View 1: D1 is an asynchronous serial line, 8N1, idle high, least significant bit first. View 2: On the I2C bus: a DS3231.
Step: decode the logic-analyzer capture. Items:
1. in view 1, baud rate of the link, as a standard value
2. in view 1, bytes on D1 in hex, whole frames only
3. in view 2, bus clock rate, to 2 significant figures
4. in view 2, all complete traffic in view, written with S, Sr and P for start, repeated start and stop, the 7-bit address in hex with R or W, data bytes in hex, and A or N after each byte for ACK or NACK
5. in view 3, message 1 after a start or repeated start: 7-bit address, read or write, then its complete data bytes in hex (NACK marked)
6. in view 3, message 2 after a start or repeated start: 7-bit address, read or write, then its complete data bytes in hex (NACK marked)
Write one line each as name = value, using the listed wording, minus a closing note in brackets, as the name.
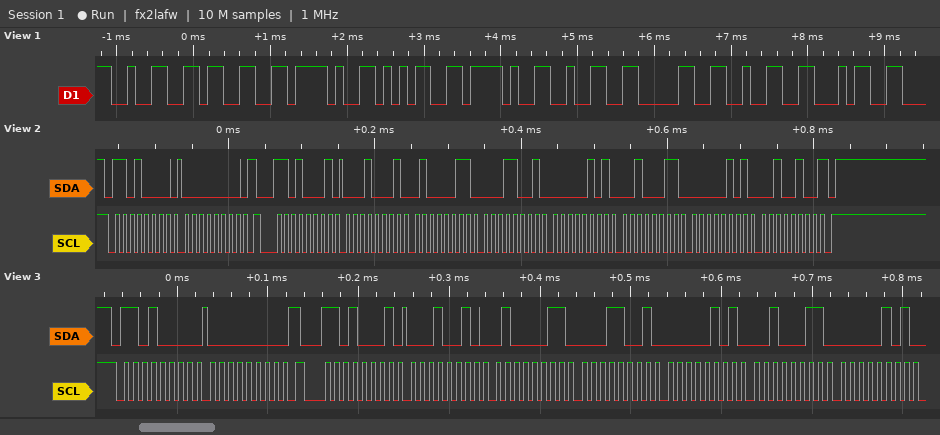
in view 1, baud rate of the link, as a standard value = 9600 baud
in view 1, bytes on D1 in hex, whole frames only = 0x32 0x33 0x2F 0x35 0x2F 0x32 0x30 0x32 0x34
in view 2, bus clock rate, to 2 significant figures = 100 kHz
in view 2, all complete traffic in view, written with S, Sr and P for start, repeated start and stop, the 7-bit address in hex with R or W, data bytes in hex, and A or N after each byte for ACK or NACK = S 68W A 00 A Sr 68R A 11 A 43 A 19 A 05 A 23 A 05 A 24 N P
in view 3, message 1 after a start or repeated start: 7-bit address, read or write, then its complete data bytes in hex = 0x68 write: 00
in view 3, message 2 after a start or repeated start: 7-bit address, read or write, then its complete data bytes in hex = 0x68 read: 12 43 19 05 23 05
